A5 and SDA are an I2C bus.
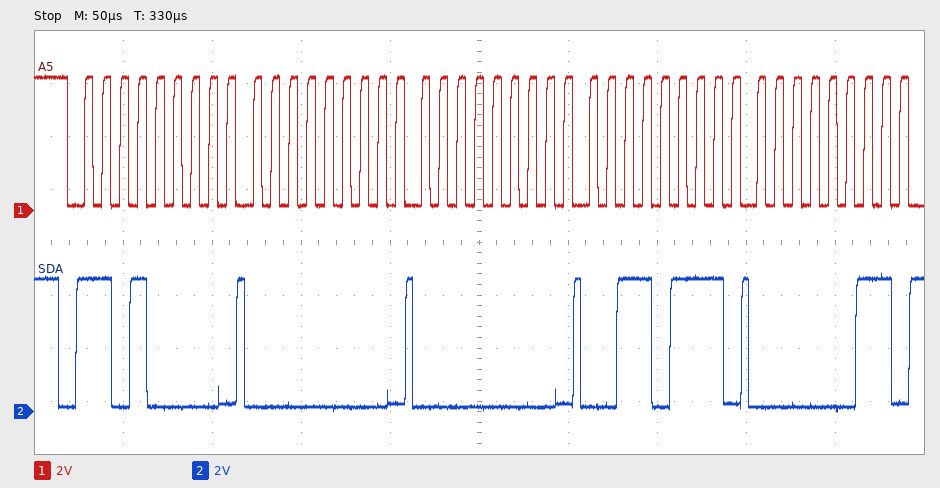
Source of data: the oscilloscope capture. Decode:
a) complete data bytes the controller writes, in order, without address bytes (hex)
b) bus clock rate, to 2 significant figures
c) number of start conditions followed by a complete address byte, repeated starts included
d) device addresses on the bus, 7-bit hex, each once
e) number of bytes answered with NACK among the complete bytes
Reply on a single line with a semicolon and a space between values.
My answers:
00 00 37 03; 100 kHz; 1; 0x68; 0
